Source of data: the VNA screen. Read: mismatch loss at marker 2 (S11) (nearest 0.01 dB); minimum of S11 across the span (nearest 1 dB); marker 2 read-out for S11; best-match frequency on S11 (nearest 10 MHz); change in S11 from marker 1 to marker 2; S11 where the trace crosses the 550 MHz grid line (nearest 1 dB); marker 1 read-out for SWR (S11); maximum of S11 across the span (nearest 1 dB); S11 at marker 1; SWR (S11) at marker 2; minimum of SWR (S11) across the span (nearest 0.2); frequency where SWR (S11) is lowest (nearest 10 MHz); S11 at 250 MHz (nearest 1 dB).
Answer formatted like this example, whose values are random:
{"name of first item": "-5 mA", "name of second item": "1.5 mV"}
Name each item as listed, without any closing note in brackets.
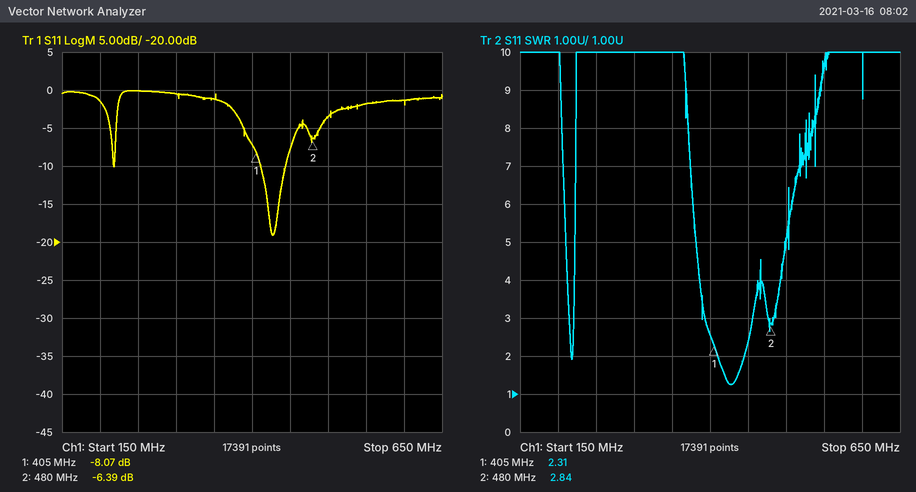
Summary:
{"mismatch loss at marker 2 (S11)": "1.13 dB", "minimum of S11 across the span": "-19 dB", "marker 2 read-out for S11": "-6.39 dB", "best-match frequency on S11": "430 MHz", "change in S11 from marker 1 to marker 2": "1.68 dB", "S11 where the trace crosses the 550 MHz grid line": "-2 dB", "marker 1 read-out for SWR": "2.31", "maximum of S11 across the span": "0 dB", "S11 at marker 1": "-8.07 dB", "SWR (S11) at marker 2": "2.84", "minimum of SWR (S11) across the span": "1.2", "frequency where SWR (S11) is lowest": "430 MHz", "S11 at 250 MHz": "0 dB"}
